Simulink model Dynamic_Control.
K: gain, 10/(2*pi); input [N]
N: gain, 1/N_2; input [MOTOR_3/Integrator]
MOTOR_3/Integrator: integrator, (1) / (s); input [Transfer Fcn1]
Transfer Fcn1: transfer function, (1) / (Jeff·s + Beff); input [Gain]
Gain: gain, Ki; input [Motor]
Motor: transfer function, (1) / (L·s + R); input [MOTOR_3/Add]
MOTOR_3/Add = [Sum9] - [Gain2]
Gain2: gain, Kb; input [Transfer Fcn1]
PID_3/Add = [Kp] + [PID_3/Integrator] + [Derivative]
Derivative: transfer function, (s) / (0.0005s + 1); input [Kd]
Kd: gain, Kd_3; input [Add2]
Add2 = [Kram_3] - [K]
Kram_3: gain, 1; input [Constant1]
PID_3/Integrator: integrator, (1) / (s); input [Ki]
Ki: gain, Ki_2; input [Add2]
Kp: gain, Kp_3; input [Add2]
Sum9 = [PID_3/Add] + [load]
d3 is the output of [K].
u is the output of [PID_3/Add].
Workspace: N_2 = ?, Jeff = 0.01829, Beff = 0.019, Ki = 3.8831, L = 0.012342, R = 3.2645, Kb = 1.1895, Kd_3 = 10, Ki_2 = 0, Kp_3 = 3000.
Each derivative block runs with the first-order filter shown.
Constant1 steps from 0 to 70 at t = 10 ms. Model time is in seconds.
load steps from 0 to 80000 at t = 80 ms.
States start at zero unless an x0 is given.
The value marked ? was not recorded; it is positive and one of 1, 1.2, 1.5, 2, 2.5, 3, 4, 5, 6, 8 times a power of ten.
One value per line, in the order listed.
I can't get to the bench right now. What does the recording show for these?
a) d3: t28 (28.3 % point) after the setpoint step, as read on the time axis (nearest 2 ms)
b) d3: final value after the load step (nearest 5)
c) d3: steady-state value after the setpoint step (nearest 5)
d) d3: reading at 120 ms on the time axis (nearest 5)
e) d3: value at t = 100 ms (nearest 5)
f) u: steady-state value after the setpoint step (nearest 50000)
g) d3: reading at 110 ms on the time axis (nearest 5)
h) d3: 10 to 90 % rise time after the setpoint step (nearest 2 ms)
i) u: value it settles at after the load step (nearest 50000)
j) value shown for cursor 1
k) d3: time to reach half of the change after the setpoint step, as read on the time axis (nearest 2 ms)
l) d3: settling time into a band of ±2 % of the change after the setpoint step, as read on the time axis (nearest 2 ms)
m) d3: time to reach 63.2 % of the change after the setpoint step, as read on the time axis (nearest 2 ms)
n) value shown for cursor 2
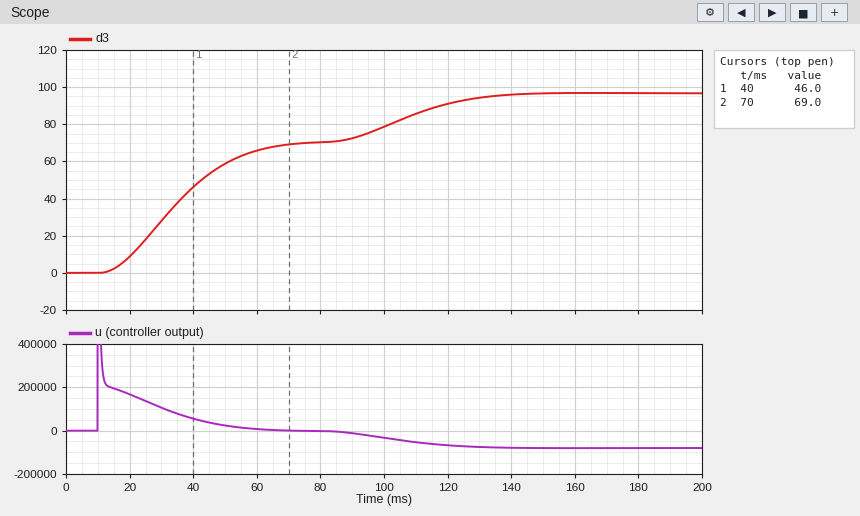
26 ms
95
70
90
80
0
85
36 ms
-100000
46.0
34 ms
68 ms
38 ms
69.0
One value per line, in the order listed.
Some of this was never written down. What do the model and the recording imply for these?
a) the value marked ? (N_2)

100
